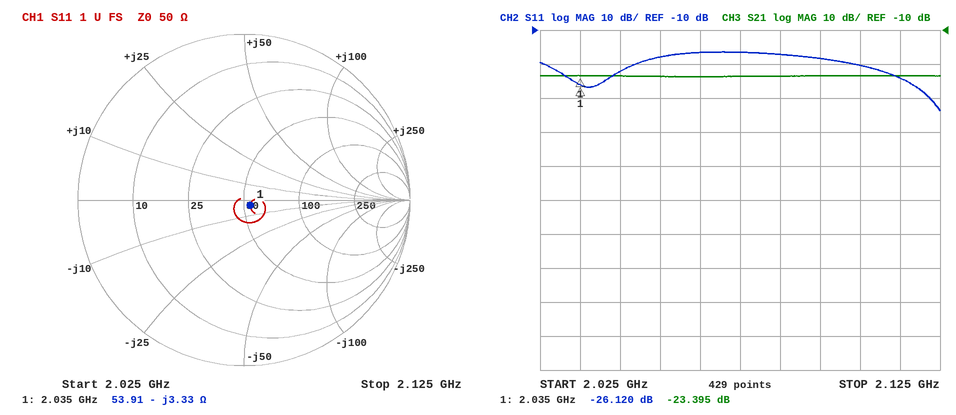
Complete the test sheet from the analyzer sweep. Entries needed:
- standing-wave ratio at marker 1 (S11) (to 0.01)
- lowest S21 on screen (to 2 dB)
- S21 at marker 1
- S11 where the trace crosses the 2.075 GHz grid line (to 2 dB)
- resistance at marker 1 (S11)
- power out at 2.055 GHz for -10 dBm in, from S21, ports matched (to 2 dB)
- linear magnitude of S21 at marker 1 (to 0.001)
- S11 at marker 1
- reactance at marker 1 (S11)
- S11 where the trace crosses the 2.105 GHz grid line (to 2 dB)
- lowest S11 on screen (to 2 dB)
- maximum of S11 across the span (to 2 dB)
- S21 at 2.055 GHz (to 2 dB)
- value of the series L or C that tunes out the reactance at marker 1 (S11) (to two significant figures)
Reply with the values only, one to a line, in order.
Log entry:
1.10
-24 dB
-23.395 dB
-16 dB
53.91 Ω
-34 dBm
0.068
-26.120 dB
-3.33 Ω
-20 dB
-34 dB
-16 dB
-24 dB
260 pH
